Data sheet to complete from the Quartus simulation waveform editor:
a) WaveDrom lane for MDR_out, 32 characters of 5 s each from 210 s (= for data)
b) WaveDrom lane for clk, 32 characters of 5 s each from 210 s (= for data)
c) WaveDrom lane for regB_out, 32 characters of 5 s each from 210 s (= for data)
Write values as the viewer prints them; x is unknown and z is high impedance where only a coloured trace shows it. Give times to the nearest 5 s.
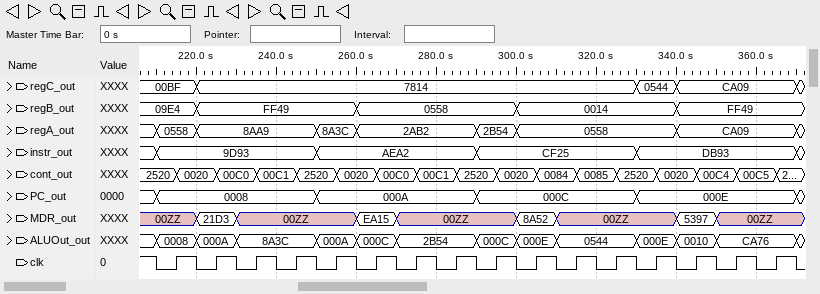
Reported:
{name: 'MDR_out', wave: '=.=.=.....=.=.....=.=.....=.=...', data: '00ZZ 21D3 00ZZ EA15 00ZZ 8A52 00ZZ 5397 00ZZ'}
{name: 'clk', wave: '01010101010101010101010101010101'}
{name: 'regB_out', wave: '=.=.......=.......=.......=.....', data: '09E4 FF49 0558 0014 FF49'}
